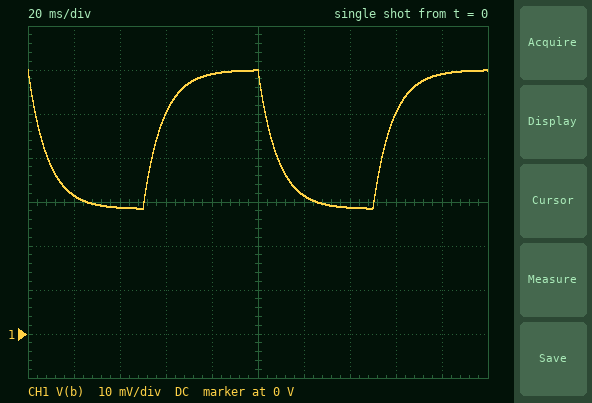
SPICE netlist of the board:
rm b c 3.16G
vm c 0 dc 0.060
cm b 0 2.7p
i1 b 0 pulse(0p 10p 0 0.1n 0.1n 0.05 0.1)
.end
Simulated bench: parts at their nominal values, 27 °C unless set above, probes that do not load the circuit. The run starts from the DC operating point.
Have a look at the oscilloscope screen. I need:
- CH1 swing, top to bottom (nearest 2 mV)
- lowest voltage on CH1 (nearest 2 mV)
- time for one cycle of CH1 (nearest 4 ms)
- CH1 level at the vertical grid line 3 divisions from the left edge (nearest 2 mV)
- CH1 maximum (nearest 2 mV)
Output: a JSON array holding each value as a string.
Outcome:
["32 mV", "28 mV", "100 ms", "50 mV", "60 mV"]
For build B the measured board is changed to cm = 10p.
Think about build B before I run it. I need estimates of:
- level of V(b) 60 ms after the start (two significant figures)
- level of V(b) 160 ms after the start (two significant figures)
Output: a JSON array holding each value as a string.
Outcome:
["42 mV", "41 mV"]
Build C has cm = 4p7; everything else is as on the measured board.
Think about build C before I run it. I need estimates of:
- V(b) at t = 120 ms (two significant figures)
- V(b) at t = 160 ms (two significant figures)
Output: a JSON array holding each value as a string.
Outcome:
["36 mV", "44 mV"]
